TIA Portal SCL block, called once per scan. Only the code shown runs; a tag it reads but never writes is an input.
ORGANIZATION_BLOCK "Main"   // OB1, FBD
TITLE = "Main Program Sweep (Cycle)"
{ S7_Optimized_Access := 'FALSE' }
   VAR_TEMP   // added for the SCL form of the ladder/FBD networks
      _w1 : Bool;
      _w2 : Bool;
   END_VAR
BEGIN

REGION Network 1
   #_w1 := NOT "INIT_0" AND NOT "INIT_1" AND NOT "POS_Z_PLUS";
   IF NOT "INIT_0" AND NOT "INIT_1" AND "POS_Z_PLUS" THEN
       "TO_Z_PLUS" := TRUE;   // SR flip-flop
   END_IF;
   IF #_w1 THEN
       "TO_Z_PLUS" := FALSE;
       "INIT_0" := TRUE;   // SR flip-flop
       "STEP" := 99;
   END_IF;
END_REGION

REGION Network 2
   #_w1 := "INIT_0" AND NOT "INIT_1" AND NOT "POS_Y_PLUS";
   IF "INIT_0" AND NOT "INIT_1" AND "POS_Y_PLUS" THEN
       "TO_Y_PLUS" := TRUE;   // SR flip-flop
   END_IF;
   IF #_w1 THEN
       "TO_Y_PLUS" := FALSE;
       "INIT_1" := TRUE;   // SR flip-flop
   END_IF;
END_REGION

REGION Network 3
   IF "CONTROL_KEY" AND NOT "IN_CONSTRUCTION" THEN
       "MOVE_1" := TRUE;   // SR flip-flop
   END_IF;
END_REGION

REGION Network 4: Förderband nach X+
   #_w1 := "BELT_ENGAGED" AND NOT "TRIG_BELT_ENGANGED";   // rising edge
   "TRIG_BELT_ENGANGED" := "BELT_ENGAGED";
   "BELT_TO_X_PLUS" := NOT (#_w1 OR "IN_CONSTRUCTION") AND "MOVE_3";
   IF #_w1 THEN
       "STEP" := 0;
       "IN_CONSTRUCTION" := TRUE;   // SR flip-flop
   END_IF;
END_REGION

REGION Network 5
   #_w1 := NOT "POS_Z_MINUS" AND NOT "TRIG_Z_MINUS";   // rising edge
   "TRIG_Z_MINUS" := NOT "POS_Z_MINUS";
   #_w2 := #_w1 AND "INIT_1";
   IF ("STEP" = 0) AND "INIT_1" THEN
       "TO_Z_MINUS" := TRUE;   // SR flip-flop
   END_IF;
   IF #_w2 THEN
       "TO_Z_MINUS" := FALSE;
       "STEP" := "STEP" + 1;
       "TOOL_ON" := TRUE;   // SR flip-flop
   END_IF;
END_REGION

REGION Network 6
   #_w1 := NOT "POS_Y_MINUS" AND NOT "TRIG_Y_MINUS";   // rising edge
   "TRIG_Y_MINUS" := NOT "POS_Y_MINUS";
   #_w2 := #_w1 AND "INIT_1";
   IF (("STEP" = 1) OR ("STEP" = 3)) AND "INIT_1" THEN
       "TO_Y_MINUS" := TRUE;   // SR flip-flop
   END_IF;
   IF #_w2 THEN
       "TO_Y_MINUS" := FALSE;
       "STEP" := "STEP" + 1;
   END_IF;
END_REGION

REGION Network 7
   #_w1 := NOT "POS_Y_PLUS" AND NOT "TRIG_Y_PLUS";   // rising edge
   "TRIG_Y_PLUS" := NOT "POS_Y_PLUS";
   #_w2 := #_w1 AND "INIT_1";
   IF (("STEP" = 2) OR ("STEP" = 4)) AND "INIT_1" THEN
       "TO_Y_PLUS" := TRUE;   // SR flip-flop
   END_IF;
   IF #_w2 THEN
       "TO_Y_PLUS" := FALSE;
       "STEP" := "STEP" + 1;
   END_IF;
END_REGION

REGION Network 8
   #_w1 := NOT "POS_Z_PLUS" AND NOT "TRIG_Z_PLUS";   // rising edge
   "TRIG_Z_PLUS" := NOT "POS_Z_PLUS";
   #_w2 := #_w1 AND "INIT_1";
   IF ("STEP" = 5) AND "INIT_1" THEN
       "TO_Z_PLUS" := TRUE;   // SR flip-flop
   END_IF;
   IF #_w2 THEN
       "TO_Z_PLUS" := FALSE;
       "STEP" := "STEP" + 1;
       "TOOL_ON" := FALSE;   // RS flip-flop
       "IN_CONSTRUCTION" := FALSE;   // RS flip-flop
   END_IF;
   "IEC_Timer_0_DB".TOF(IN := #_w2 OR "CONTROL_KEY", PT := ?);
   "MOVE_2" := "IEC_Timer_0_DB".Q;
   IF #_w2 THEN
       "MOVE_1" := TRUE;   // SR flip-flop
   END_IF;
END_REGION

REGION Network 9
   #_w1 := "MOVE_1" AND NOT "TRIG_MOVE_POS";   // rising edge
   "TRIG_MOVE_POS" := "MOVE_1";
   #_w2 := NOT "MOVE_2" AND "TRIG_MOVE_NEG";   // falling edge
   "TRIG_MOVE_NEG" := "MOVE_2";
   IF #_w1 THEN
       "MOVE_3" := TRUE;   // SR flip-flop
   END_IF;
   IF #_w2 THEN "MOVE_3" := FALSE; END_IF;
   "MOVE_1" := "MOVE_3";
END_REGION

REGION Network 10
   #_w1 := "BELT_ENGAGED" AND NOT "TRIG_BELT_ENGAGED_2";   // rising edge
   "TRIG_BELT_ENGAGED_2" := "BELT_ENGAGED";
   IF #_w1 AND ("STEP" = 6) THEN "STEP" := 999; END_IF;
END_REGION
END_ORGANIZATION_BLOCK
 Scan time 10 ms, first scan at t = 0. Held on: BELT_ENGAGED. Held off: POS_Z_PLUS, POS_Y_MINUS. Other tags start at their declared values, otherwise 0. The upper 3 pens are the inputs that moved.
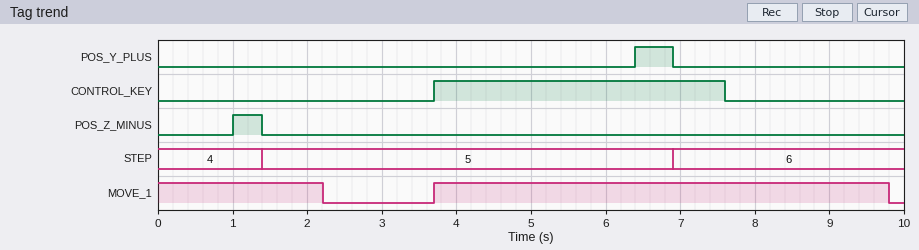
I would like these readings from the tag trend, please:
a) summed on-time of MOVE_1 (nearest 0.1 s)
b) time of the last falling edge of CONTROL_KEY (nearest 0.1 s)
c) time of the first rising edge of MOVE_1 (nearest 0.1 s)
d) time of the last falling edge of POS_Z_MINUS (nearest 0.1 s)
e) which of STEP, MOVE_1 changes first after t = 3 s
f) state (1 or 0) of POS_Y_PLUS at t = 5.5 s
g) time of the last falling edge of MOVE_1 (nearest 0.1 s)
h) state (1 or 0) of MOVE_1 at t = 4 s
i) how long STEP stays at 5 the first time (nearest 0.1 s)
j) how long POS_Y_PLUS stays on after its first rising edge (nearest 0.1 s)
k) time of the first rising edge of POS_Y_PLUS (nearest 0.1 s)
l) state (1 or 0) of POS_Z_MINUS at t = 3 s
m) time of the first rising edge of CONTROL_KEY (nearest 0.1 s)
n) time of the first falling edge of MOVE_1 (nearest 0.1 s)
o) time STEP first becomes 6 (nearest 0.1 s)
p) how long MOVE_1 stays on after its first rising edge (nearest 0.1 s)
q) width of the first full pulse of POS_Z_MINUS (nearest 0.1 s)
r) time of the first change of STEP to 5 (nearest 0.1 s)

8.3 s
7.6 s
3.7 s
1.4 s
MOVE_1
0
9.8 s
1
5.5 s
0.5 s
6.4 s
0
3.7 s
2.2 s
6.9 s
6.1 s
0.4 s
1.4 s
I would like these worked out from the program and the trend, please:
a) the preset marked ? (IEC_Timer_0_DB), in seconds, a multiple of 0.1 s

2.2 s
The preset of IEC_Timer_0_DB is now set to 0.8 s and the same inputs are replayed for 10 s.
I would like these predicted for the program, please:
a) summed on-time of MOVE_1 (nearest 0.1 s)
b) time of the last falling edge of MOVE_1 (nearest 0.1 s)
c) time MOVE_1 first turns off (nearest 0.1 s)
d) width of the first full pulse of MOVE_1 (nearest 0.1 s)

5.5 s
8.4 s
0.8 s
4.7 s
